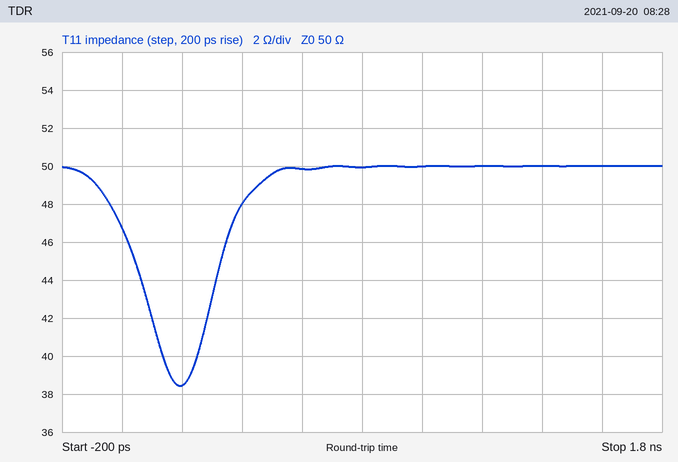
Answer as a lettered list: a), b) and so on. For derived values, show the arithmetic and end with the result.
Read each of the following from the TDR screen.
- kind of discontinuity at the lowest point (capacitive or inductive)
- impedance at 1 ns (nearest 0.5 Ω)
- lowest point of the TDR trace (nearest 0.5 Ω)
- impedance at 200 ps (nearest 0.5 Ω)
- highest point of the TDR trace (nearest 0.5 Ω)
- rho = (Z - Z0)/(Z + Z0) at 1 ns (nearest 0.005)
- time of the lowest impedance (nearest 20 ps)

a) capacitive
b) 50.0 Ω
c) 38.5 Ω
d) 38.5 Ω
e) 50.0 Ω
f) (50 − 50)/(50 + 50) ≈ 0.000
g) 200 ps
